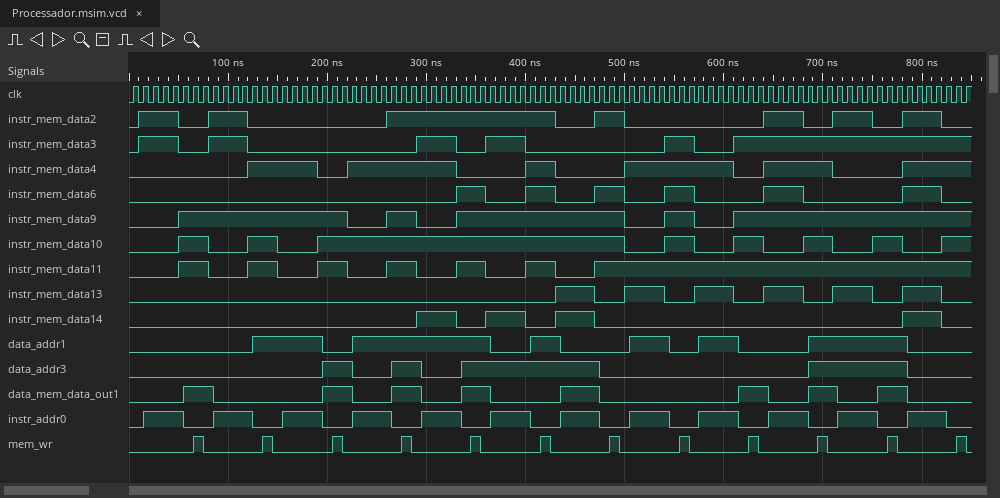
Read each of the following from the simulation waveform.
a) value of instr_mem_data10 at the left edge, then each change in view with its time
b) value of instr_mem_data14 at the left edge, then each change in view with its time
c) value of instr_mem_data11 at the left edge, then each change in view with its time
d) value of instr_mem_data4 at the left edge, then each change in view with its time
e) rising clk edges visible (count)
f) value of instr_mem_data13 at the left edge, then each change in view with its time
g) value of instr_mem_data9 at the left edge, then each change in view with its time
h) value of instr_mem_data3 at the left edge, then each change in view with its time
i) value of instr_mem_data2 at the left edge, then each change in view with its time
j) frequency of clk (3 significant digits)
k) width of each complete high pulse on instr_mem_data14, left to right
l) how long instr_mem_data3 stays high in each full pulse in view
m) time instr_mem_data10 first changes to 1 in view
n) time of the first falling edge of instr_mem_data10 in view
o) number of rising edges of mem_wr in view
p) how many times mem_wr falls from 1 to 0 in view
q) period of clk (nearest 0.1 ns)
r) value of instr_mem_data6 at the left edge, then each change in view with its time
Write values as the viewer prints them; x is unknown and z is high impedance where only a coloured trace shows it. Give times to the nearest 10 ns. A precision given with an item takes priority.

0, 1 at 50 ns, 0 at 80 ns, 1 at 120 ns, 0 at 150 ns, 1 at 190 ns, 0 at 500 ns, 1 at 540 ns, 0 at 570 ns, 1 at 610 ns, 0 at 640 ns, 1 at 680 ns, 0 at 710 ns, 1 at 750 ns, 0 at 780 ns, 1 at 820 ns
0, 1 at 290 ns, 0 at 330 ns, 1 at 360 ns, 0 at 400 ns, 1 at 430 ns, 0 at 470 ns, 1 at 780 ns, 0 at 820 ns
0, 1 at 50 ns, 0 at 80 ns, 1 at 120 ns, 0 at 150 ns, 1 at 190 ns, 0 at 220 ns, 1 at 260 ns, 0 at 290 ns, 1 at 330 ns, 0 at 360 ns, 1 at 400 ns, 0 at 430 ns, 1 at 470 ns
0, 1 at 120 ns, 0 at 190 ns, 1 at 220 ns, 0 at 330 ns, 1 at 400 ns, 0 at 430 ns, 1 at 500 ns, 0 at 610 ns, 1 at 640 ns, 0 at 710 ns, 1 at 780 ns
85
0, 1 at 430 ns, 0 at 470 ns, 1 at 500 ns, 0 at 540 ns, 1 at 570 ns, 0 at 610 ns, 1 at 640 ns, 0 at 680 ns, 1 at 710 ns, 0 at 750 ns, 1 at 780 ns, 0 at 820 ns
0, 1 at 50 ns, 0 at 220 ns, 1 at 260 ns, 0 at 290 ns, 1 at 330 ns, 0 at 500 ns, 1 at 540 ns, 0 at 570 ns, 1 at 610 ns
0, 1 at 10 ns, 0 at 50 ns, 1 at 80 ns, 0 at 120 ns, 1 at 290 ns, 0 at 330 ns, 1 at 360 ns, 0 at 400 ns, 1 at 540 ns, 0 at 570 ns, 1 at 610 ns
0, 1 at 10 ns, 0 at 50 ns, 1 at 80 ns, 0 at 120 ns, 1 at 260 ns, 0 at 430 ns, 1 at 470 ns, 0 at 500 ns, 1 at 640 ns, 0 at 680 ns, 1 at 710 ns, 0 at 750 ns, 1 at 780 ns, 0 at 820 ns
100 MHz
40 ns, 40 ns, 40 ns, 40 ns
40 ns, 40 ns, 40 ns, 40 ns, 30 ns
50 ns
80 ns
12
12
10 ns
0, 1 at 330 ns, 0 at 360 ns, 1 at 400 ns, 0 at 430 ns, 1 at 470 ns, 0 at 500 ns, 1 at 540 ns, 0 at 570 ns, 1 at 640 ns, 0 at 680 ns, 1 at 780 ns, 0 at 820 ns
